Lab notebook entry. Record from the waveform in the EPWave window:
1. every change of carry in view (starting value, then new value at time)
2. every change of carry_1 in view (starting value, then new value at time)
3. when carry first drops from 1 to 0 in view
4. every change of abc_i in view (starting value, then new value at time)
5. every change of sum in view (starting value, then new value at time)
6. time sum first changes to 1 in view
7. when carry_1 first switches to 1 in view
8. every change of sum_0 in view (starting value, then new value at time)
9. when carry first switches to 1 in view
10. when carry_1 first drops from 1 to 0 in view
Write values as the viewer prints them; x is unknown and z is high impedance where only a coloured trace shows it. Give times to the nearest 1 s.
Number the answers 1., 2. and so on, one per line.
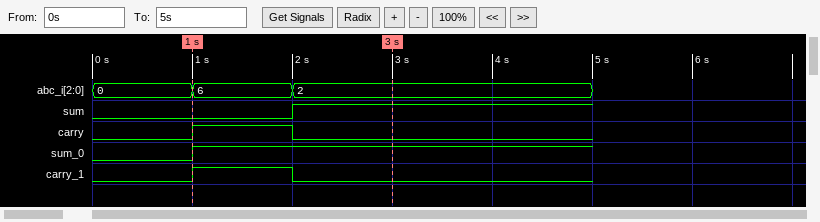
1. 0, 1 at 1 s, 0 at 2 s
2. 0, 1 at 1 s, 0 at 2 s
3. 2 s
4. 0, 6 at 1 s, 2 at 2 s
5. 0, 1 at 2 s
6. 2 s
7. 1 s
8. 0, 1 at 1 s
9. 1 s
10. 2 s
